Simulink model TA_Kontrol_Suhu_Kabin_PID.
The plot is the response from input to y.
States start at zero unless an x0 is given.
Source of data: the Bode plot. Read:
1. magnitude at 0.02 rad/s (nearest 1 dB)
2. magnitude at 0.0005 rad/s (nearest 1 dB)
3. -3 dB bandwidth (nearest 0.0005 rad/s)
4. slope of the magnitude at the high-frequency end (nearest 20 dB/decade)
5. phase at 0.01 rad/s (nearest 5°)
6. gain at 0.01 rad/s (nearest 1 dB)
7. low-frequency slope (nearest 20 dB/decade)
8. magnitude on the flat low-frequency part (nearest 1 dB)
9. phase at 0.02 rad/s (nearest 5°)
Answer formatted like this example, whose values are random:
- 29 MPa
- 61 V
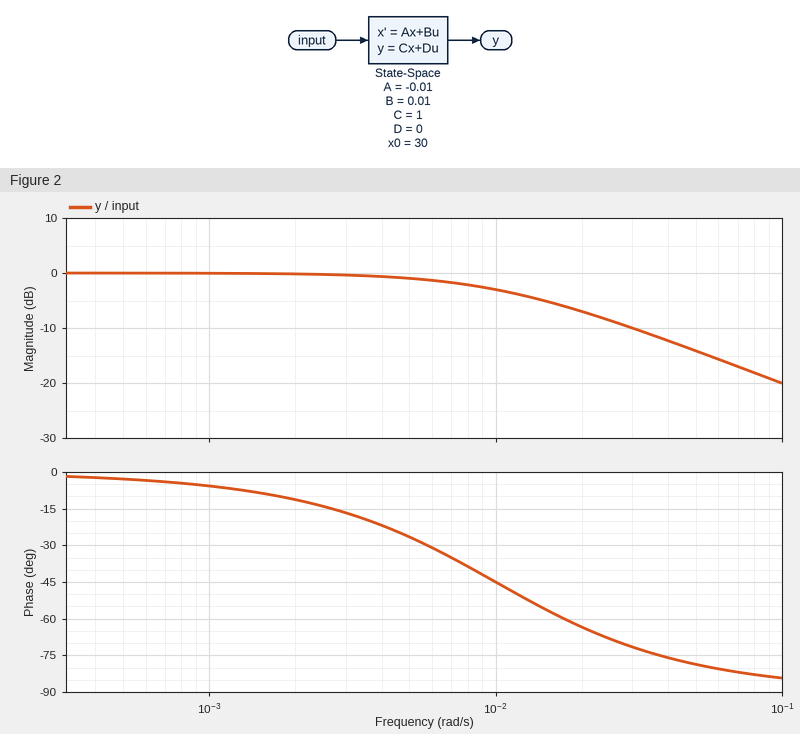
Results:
- -7 dB
- 0 dB
- 0.0100 rad/s
- -20 dB/decade
- -45°
- -3 dB
- 0 dB/decade
- 0 dB
- -65°
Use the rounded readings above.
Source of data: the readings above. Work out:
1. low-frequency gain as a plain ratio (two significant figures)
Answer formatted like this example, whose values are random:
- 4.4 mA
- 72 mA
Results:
- 1.0
